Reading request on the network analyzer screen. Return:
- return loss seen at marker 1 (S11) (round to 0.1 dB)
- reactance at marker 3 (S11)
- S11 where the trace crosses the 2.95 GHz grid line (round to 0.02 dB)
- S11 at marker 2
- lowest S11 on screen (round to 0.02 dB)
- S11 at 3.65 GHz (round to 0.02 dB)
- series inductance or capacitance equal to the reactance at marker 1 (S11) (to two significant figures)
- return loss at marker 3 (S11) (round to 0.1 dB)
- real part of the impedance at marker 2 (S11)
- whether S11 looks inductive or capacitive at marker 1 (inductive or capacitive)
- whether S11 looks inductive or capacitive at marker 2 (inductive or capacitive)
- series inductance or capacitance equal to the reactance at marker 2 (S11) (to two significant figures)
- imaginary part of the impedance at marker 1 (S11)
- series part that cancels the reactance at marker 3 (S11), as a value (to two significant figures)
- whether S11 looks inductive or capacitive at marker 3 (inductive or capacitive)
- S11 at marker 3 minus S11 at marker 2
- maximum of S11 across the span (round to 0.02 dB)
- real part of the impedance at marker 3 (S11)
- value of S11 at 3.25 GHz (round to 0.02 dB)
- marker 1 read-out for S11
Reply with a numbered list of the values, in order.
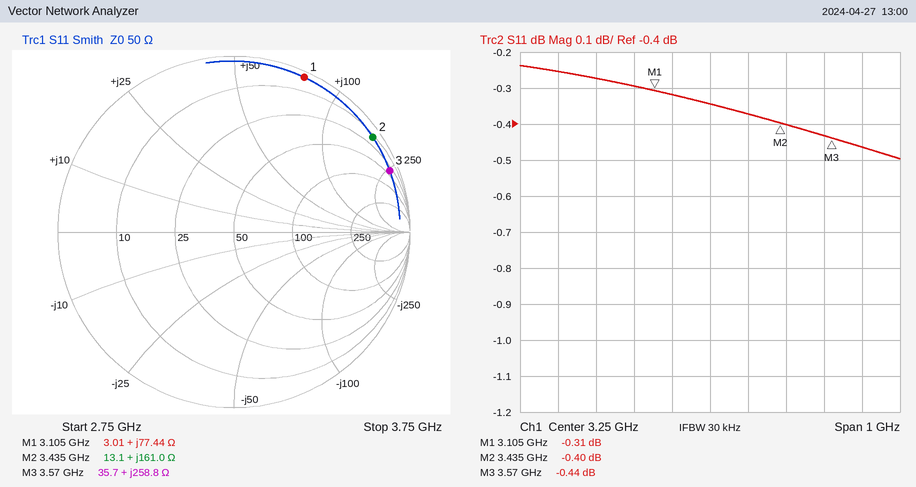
1. 0.3 dB
2. +258.8 Ω
3. -0.28 dB
4. -0.40 dB
5. -0.50 dB
6. -0.46 dB
7. 4.0 nH
8. 0.4 dB
9. 13.1 Ω
10. inductive
11. inductive
12. 7.5 nH
13. +77.44 Ω
14. 170 fF
15. inductive
16. -0.04 dB
17. -0.24 dB
18. 35.7 Ω
19. -0.34 dB
20. -0.31 dB
